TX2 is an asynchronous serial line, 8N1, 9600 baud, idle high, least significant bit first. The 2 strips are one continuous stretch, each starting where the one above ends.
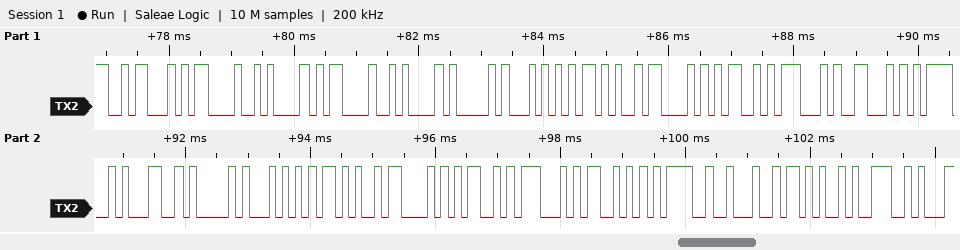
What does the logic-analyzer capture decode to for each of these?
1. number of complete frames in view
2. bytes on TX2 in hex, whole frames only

25
1A 0D 0A 0D 0A 41 54 2B 43 4D 47 46 3D 31 41 54 2B 43 4D 47 53 3D 22 2B 39
